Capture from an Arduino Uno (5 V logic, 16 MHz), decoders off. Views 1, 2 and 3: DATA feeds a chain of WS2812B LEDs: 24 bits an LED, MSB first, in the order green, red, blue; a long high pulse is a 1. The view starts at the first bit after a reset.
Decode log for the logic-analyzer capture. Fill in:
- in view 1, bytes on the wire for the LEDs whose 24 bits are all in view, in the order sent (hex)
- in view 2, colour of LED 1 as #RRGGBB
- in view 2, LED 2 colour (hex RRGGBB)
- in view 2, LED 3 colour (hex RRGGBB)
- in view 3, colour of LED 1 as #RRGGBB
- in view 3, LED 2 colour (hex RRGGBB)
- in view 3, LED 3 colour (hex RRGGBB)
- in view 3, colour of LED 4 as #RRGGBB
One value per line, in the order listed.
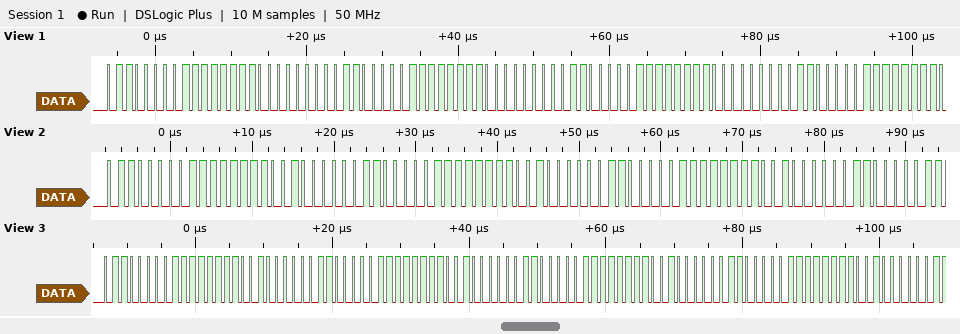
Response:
60 FF 00 60 FF 00 60 FF 00
#FF6020
#FF6020
#FF6020
#FF6020
#FF6020
#FF6020
#FF6020
